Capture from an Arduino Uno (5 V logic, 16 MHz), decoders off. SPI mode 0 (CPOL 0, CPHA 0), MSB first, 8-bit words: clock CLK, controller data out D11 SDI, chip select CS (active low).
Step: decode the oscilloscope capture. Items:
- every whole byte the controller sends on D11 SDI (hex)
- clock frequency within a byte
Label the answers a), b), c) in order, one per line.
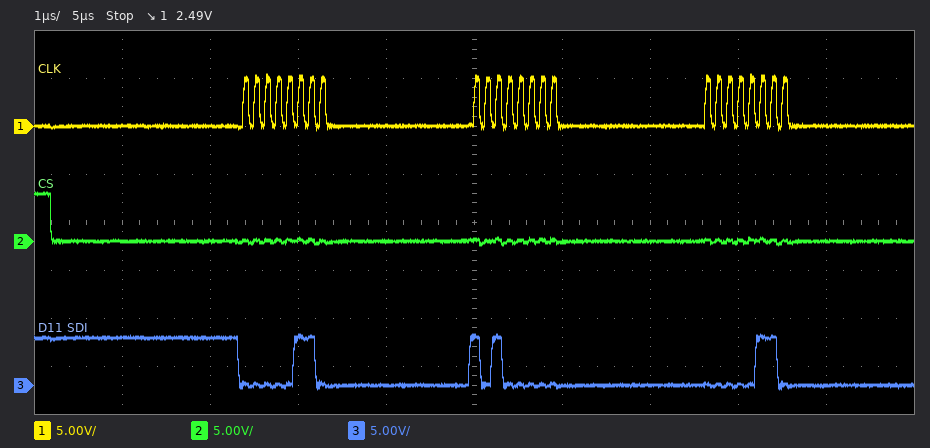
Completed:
a) 06 A0 06
b) 8 MHz
